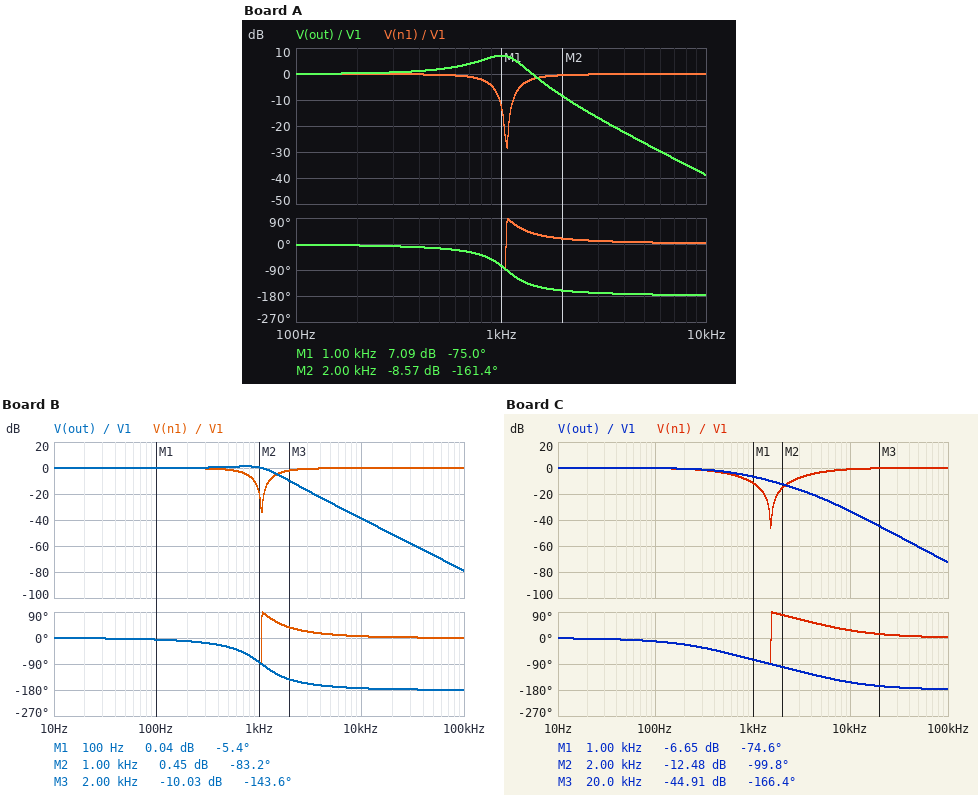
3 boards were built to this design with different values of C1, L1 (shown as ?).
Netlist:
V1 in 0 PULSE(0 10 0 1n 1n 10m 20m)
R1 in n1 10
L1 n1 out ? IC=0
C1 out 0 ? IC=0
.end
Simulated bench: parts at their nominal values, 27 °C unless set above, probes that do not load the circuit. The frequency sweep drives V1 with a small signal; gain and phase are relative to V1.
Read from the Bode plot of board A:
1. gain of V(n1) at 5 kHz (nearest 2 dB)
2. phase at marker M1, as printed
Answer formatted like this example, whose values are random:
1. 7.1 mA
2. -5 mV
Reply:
1. 0 dB
2. -75.0 deg
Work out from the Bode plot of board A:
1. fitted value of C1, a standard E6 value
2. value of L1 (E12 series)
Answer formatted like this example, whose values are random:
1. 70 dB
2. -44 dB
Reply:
1. 6.8 µF
2. 3.3 mH
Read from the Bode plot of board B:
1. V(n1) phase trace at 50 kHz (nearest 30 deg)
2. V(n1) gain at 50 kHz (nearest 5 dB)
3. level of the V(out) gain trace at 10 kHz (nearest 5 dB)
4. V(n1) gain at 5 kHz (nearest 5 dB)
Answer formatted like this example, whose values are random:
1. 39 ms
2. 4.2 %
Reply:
1. 0 deg
2. 0 dB
3. -40 dB
4. 0 dB
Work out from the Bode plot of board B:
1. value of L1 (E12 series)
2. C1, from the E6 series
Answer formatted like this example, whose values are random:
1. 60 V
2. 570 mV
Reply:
1. 1.5 mH
2. 15 µF
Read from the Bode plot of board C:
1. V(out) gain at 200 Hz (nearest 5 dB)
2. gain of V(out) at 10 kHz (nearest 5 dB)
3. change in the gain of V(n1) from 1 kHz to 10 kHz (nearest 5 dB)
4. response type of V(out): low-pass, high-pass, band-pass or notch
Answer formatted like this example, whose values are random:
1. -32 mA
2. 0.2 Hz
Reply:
1. 0 dB
2. -35 dB
3. 10 dB
4. low-pass
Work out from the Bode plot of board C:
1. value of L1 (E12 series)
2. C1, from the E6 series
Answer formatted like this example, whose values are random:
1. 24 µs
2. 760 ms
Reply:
1. 330 µH
2. 33 µF
